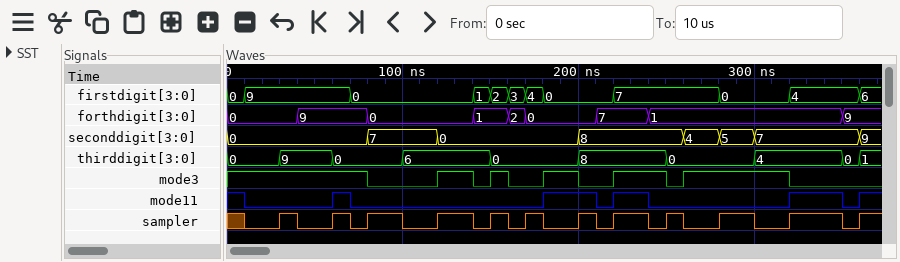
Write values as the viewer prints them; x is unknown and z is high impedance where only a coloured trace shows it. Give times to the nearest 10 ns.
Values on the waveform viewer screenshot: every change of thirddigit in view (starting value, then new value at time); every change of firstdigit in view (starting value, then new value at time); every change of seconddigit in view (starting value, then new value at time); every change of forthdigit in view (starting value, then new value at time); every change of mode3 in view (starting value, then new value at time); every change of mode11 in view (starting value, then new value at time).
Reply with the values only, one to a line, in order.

0, 9 at 30 ns, 0 at 60 ns, 6 at 100 ns, 0 at 150 ns, 8 at 200 ns, 0 at 250 ns, 4 at 300 ns, 0 at 350 ns, 1 at 360 ns
0, 9 at 10 ns, 0 at 70 ns, 1 at 140 ns, 2 at 150 ns, 3 at 160 ns, 4 at 170 ns, 0 at 180 ns, 7 at 220 ns, 0 at 280 ns, 4 at 320 ns, 6 at 360 ns
0, 7 at 80 ns, 0 at 120 ns, 8 at 200 ns, 4 at 260 ns, 5 at 280 ns, 7 at 300 ns, 9 at 360 ns
0, 9 at 40 ns, 0 at 80 ns, 1 at 140 ns, 2 at 160 ns, 0 at 170 ns, 7 at 210 ns, 1 at 240 ns, 9 at 350 ns
1, 0 at 80 ns, 1 at 120 ns, 0 at 140 ns, 1 at 150 ns, 0 at 160 ns, 1 at 180 ns, 0 at 200 ns, 1 at 220 ns, 0 at 250 ns, 1 at 260 ns, 0 at 320 ns
1, 0 at 10 ns, 1 at 60 ns, 0 at 70 ns, 1 at 180 ns, 0 at 210 ns, 1 at 220 ns, 0 at 240 ns, 1 at 320 ns, 0 at 350 ns, 1 at 360 ns
